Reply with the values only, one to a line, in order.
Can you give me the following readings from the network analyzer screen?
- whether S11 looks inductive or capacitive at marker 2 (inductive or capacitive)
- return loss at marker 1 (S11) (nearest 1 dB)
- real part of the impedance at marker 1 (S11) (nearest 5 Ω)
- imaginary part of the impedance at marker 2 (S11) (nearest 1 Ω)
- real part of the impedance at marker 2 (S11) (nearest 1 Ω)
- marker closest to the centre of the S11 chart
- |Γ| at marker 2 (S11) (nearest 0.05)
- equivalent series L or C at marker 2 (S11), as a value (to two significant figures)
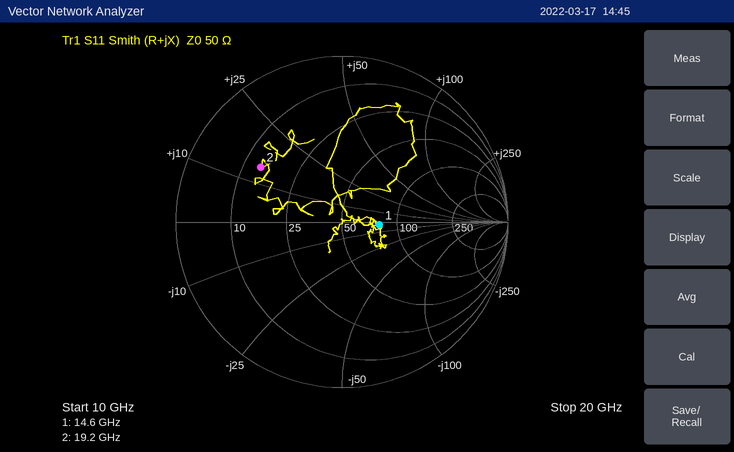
inductive
13 dB
80 Ω
+14 Ω
14 Ω
marker 1
0.60
120 pH
